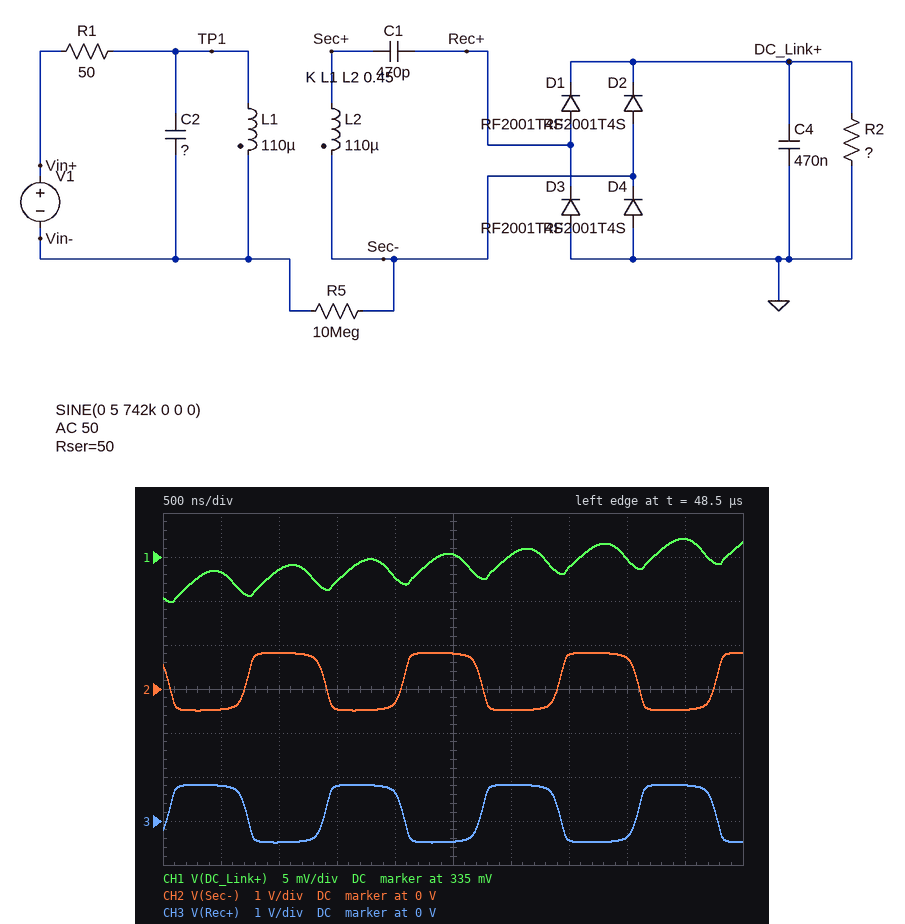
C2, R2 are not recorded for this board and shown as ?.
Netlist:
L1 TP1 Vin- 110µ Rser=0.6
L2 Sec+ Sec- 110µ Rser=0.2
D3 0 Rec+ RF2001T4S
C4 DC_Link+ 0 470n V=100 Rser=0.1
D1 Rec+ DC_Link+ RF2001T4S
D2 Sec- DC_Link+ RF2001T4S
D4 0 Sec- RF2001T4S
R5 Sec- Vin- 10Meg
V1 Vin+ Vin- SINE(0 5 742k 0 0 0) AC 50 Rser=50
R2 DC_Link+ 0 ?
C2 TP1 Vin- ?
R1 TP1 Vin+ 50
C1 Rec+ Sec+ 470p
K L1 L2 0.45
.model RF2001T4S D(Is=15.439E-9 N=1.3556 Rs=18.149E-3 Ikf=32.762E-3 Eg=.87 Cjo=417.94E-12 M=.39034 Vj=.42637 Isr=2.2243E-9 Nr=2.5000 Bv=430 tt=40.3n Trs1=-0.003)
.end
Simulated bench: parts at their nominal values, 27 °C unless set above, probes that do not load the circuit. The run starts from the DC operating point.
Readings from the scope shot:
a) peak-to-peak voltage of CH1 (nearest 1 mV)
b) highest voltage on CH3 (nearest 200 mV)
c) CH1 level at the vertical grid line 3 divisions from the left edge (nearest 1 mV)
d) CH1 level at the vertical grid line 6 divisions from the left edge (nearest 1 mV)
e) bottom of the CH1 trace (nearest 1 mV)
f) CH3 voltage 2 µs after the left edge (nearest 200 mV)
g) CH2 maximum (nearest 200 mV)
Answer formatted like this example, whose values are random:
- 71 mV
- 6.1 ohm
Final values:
- 7 mV
- 800 mV
- 332 mV
- 335 mV
- 330 mV
- 600 mV
- 800 mV
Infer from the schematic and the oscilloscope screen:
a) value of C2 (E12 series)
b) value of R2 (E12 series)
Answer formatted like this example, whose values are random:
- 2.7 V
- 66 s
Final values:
- 1.2 nF
- 68 Ω
